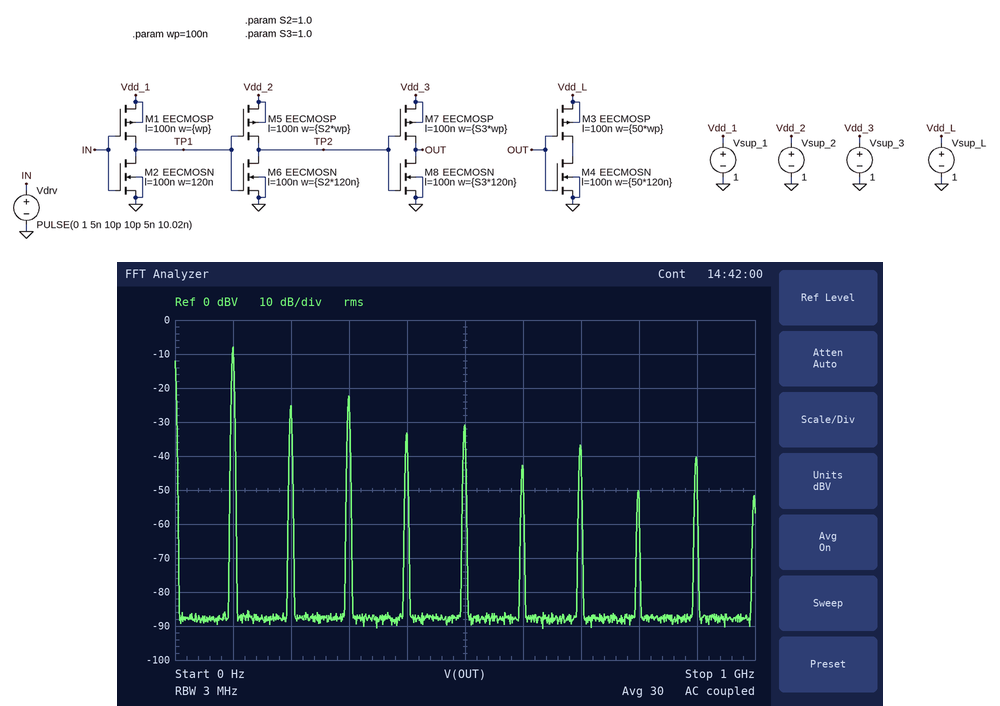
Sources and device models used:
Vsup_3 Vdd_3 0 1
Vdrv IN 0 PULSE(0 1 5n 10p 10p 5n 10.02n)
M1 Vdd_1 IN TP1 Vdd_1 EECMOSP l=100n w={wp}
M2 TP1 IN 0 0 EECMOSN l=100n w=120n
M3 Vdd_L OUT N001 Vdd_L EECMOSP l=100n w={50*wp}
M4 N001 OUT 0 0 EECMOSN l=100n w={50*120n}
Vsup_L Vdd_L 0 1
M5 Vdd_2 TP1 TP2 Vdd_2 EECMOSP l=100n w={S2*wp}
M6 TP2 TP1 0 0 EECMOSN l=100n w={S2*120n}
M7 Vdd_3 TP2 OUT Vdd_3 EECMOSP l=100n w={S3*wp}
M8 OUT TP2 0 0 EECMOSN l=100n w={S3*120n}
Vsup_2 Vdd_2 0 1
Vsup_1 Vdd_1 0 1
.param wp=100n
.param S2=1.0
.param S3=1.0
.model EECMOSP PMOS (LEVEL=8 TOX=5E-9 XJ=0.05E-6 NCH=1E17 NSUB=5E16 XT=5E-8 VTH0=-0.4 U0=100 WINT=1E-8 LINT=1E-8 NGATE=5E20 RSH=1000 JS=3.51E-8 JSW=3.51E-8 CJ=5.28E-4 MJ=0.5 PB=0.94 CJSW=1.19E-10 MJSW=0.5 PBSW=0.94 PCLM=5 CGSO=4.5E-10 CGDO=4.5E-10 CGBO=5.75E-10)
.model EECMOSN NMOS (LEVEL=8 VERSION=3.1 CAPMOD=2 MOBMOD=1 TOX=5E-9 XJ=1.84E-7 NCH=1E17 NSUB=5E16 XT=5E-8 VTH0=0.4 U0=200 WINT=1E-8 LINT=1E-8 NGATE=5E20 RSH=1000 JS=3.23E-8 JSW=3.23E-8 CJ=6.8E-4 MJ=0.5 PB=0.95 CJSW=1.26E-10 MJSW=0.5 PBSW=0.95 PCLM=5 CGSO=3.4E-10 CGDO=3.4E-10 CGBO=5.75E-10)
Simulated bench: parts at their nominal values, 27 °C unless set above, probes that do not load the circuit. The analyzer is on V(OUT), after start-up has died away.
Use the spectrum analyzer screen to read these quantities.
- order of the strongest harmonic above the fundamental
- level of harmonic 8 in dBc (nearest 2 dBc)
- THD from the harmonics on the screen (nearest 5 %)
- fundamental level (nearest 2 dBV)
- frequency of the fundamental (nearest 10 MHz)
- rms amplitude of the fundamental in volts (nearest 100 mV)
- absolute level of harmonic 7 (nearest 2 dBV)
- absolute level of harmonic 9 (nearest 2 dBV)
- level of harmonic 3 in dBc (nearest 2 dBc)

3
-42 dBc
25 %
-8 dBV
100 MHz
400 mV
-36 dBV
-40 dBV
-14 dBc
